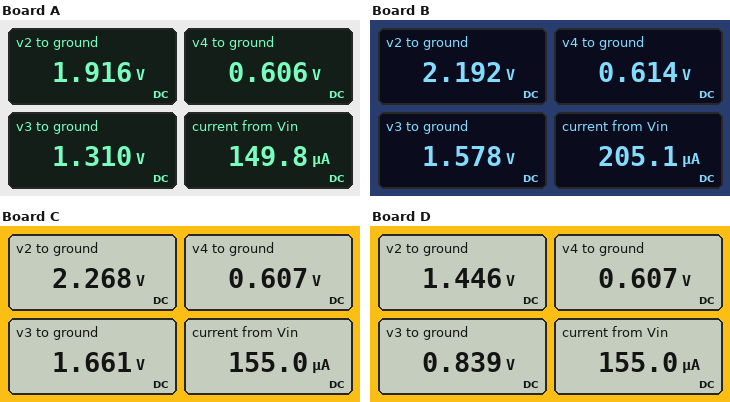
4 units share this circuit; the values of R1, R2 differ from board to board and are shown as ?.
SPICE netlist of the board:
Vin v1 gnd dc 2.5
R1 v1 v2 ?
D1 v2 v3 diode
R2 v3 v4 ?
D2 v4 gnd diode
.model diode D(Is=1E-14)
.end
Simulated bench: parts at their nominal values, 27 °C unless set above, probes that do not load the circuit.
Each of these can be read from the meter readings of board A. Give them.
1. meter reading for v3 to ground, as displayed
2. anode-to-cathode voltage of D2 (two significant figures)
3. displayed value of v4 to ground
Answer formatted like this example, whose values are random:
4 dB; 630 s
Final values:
1.310 V; 610 mV; 0.606 V
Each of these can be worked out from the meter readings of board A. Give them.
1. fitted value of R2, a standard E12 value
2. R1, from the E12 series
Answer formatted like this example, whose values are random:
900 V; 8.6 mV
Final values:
4.7 kΩ; 3.9 kΩ
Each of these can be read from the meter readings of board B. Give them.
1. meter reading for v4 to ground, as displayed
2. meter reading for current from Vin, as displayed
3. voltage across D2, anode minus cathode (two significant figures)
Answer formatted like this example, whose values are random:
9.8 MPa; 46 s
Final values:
0.614 V; 205.1 µA; 610 mV
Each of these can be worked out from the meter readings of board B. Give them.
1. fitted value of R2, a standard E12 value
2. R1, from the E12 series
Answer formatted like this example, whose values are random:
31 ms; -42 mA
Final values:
4.7 kΩ; 1.5 kΩ
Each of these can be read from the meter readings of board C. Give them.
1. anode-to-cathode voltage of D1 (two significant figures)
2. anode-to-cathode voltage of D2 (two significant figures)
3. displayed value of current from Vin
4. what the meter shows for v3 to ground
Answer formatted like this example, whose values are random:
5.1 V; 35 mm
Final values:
610 mV; 610 mV; 155.0 µA; 1.661 V
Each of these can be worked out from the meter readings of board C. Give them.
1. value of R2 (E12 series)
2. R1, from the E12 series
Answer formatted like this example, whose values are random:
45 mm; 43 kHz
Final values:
6.8 kΩ; 1.5 kΩ
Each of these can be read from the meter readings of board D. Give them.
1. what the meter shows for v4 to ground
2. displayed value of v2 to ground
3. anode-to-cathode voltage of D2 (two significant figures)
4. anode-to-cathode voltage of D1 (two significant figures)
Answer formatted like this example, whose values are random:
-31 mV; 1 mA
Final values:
0.607 V; 1.446 V; 610 mV; 610 mV
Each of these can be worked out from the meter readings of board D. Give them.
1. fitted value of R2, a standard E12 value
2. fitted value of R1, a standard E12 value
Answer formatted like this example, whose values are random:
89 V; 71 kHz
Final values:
1.5 kΩ; 6.8 kΩ
